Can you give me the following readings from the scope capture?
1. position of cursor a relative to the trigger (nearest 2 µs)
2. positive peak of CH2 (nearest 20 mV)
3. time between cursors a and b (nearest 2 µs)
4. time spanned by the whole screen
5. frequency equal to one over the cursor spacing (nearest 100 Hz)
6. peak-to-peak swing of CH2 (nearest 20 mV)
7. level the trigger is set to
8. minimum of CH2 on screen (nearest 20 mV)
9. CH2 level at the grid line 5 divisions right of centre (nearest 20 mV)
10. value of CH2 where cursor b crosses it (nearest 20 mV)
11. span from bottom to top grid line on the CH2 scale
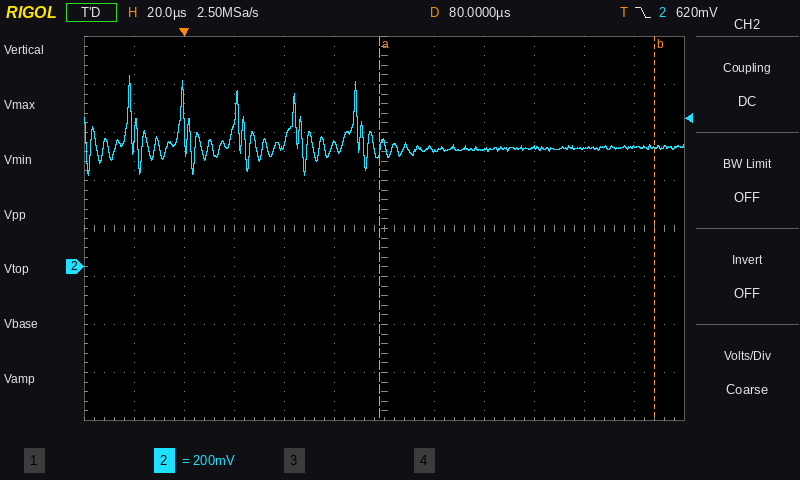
+78 µs
800 mV
110 µs
240 µs
9.1 kHz
420 mV
620 mV
380 mV
500 mV
500 mV
1.6 V
